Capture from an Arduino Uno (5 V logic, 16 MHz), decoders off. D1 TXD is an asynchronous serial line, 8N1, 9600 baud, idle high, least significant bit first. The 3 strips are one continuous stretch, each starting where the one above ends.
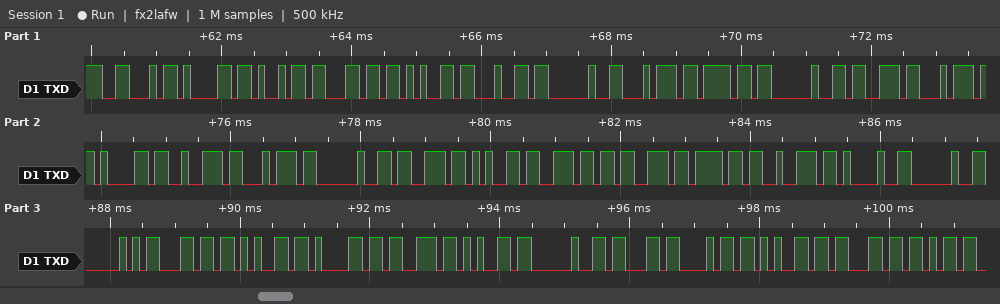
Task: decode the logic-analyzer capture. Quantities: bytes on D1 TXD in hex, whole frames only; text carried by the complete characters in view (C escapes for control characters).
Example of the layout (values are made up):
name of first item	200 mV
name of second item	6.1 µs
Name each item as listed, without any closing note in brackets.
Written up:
bytes on D1 TXD in hex, whole frames only	0x46 0x61 0x69 0x6C 0x65 0x64 0x20 0x74 0x6F 0x20 0x73 0x74 0x61 0x72 0x74 0x20 0x73 0x65 0x6E 0x73 0x6F 0x72 0x21 0x20 0x50 0x6C 0x65 0x61 0x73 0x65 0x20 0x63 0x68 0x65 0x63 0x6B
text carried by the complete characters in view	"Failed to start sensor! Please check"
